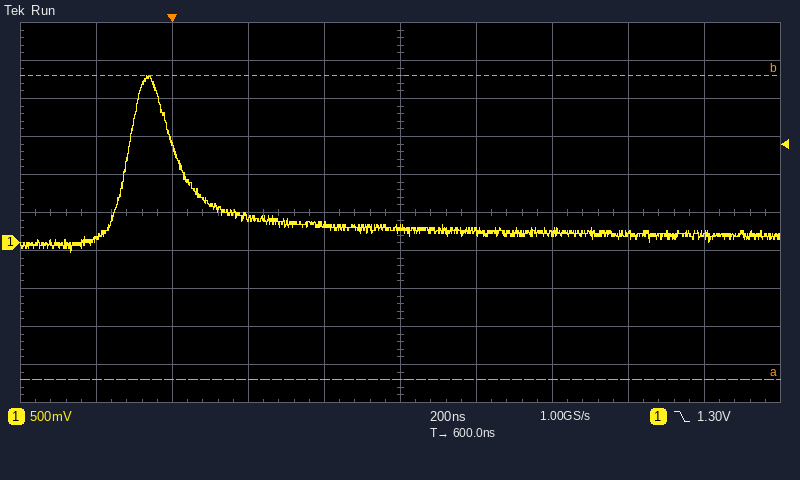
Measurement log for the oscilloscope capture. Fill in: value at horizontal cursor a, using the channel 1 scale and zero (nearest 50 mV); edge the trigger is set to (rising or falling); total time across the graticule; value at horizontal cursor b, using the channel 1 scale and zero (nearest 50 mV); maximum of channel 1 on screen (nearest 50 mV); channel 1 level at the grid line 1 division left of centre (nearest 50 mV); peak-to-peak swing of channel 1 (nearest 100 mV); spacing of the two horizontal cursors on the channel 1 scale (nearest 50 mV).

-1.80 V
falling
2 µs
2.20 V
2.20 V
250 mV
2.30 V
4.00 V
